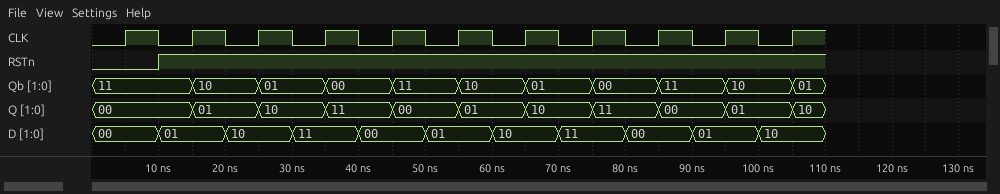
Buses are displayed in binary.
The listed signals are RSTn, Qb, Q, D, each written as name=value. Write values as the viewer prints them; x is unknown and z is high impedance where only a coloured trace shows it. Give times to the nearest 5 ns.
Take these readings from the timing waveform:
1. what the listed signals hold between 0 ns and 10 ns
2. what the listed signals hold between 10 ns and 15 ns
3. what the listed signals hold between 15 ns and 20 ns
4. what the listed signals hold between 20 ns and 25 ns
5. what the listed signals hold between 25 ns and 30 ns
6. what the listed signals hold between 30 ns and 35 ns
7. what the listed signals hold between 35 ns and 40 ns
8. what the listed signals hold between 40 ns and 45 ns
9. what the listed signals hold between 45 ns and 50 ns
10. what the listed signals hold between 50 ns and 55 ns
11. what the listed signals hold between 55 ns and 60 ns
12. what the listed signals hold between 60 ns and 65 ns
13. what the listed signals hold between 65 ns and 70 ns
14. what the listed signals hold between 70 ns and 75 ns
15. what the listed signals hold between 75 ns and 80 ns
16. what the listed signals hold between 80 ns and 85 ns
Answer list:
RSTn=0, Qb=11, Q=00, D=00
RSTn=1, Qb=11, Q=00, D=01
RSTn=1, Qb=10, Q=01, D=01
RSTn=1, Qb=10, Q=01, D=10
RSTn=1, Qb=01, Q=10, D=10
RSTn=1, Qb=01, Q=10, D=11
RSTn=1, Qb=00, Q=11, D=11
RSTn=1, Qb=00, Q=11, D=00
RSTn=1, Qb=11, Q=00, D=00
RSTn=1, Qb=11, Q=00, D=01
RSTn=1, Qb=10, Q=01, D=01
RSTn=1, Qb=10, Q=01, D=10
RSTn=1, Qb=01, Q=10, D=10
RSTn=1, Qb=01, Q=10, D=11
RSTn=1, Qb=00, Q=11, D=11
RSTn=1, Qb=00, Q=11, D=00
